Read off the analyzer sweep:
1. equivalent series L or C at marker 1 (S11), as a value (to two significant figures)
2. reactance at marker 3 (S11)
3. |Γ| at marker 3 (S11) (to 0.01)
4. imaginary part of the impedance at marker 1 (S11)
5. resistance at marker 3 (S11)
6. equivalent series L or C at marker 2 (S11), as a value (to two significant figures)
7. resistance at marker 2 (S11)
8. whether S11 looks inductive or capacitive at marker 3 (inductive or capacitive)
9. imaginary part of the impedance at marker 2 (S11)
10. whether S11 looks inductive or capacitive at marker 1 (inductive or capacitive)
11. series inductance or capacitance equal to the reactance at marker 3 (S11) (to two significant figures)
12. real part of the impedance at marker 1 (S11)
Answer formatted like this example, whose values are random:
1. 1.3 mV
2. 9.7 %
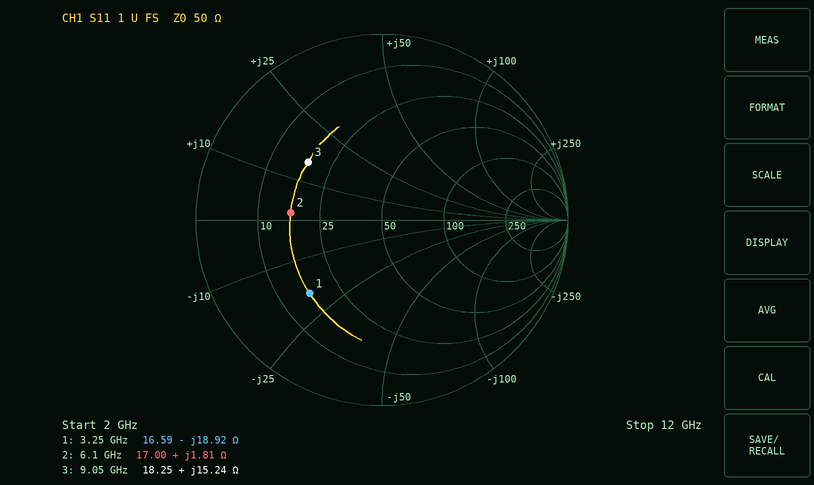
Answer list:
1. 2.6 pF
2. +15.24 Ω
3. 0.50
4. -18.92 Ω
5. 18.25 Ω
6. 47 pH
7. 17.00 Ω
8. inductive
9. +1.81 Ω
10. capacitive
11. 270 pH
12. 16.59 Ω
